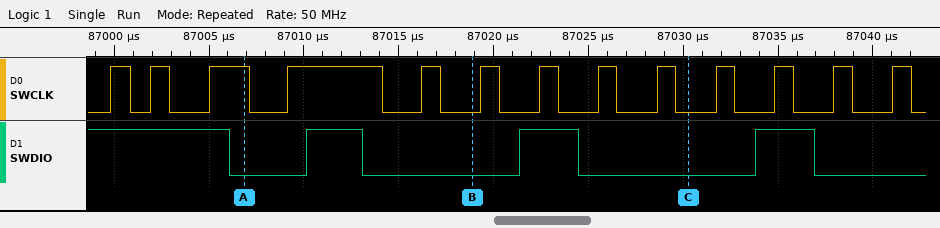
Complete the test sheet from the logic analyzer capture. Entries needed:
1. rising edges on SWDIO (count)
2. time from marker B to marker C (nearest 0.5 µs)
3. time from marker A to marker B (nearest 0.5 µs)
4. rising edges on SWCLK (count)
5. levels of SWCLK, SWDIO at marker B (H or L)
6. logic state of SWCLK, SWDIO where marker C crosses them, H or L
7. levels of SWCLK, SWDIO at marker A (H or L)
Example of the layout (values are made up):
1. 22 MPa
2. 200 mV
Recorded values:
1. 3
2. 11.5 µs
3. 12 µs
4. 13
5. SWCLK=L, SWDIO=L
6. SWCLK=L, SWDIO=L
7. SWCLK=H, SWDIO=L
